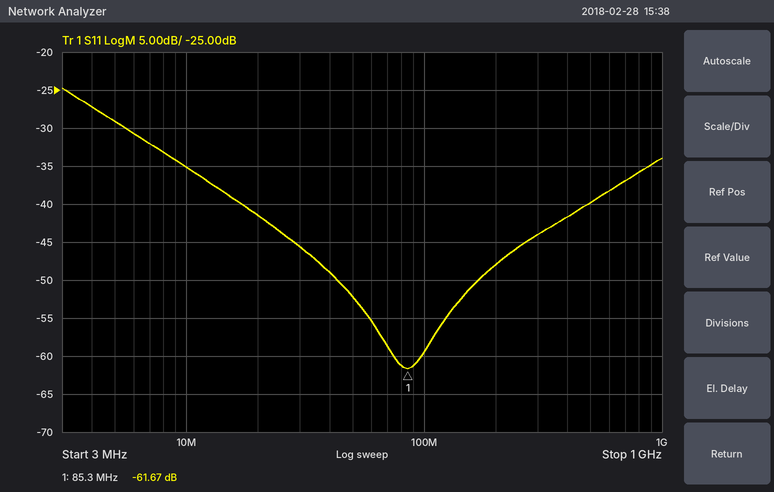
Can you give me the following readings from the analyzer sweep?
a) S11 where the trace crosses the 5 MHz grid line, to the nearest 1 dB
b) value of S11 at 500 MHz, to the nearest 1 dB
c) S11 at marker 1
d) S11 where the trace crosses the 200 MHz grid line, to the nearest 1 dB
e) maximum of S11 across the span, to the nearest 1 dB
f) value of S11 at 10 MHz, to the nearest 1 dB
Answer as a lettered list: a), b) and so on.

a) -29 dB
b) -40 dB
c) -61.67 dB
d) -48 dB
e) -25 dB
f) -35 dB
